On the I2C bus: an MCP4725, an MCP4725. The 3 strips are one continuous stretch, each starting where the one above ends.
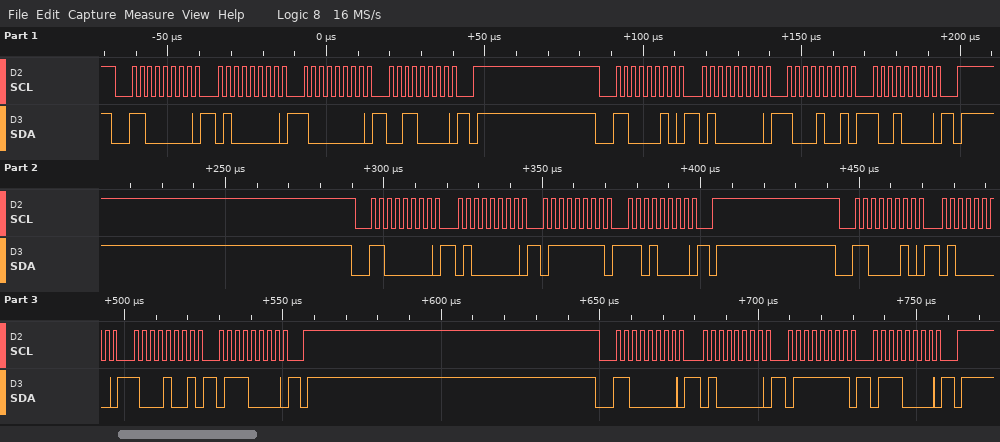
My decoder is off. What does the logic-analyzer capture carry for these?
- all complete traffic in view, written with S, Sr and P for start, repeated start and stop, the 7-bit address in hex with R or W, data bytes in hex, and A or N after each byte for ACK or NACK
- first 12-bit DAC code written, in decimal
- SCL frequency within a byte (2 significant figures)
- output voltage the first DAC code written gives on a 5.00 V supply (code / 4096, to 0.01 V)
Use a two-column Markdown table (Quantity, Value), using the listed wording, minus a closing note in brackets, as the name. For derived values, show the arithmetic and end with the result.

| Quantity | Value |
|---|---|
| all complete traffic in view, written with S, Sr and P for start, repeated start and stop, the 7-bit address in hex with R or W, data bytes in hex, and A or N after each byte for ACK or NACK | S 60W A 40 A 80 A 30 A P S 61W A 40 A 89 A 90 A P S 60W A 40 A 7F A D0 A P S 61W A 40 A 89 A 70 A P S 60W A 40 A 7F A 70 A P |
| first 12-bit DAC code written, in decimal | 2051 |
| SCL frequency within a byte | 400 kHz |
| output voltage the first DAC code written gives on a 5.00 V supply | 2051 / 4096 x 5.00 V = 2.50 V |
